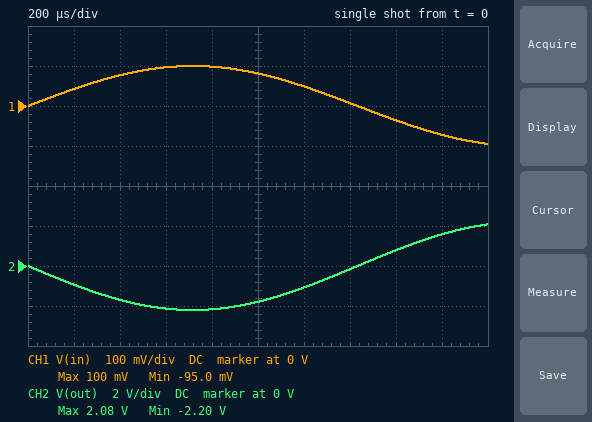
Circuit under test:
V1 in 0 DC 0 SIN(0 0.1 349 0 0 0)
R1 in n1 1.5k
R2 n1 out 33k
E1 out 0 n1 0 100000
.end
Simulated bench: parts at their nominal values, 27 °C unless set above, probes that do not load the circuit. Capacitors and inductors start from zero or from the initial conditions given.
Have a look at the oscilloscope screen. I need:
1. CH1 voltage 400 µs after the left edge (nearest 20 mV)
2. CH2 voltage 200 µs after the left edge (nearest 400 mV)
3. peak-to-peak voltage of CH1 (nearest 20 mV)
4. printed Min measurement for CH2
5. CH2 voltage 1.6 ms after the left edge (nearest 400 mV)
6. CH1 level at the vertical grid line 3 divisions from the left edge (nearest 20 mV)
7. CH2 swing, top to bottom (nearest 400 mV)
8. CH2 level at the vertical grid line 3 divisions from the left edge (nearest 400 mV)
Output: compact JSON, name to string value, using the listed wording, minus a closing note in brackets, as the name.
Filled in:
{"CH1 voltage 400 µs after the left edge": "80 mV", "CH2 voltage 200 µs after the left edge": "-800 mV", "peak-to-peak voltage of CH1": "200 mV", "printed Min measurement for CH2": "-2.20 V", "CH2 voltage 1.6 ms after the left edge": "800 mV", "CH1 level at the vertical grid line 3 divisions from the left edge": "100 mV", "CH2 swing, top to bottom": "4.4 V", "CH2 level at the vertical grid line 3 divisions from the left edge": "-2.0 V"}
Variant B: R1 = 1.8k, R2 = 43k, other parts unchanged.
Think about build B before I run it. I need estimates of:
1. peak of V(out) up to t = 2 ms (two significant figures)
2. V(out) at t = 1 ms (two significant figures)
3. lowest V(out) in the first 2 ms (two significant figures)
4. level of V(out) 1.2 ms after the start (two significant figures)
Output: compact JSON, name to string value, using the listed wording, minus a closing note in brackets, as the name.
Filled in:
{"peak of V(out) up to t = 2 ms": "2.3 V", "V(out) at t = 1 ms": "-1.9 V", "lowest V(out) in the first 2 ms": "-2.4 V", "level of V(out) 1.2 ms after the start": "-1.2 V"}
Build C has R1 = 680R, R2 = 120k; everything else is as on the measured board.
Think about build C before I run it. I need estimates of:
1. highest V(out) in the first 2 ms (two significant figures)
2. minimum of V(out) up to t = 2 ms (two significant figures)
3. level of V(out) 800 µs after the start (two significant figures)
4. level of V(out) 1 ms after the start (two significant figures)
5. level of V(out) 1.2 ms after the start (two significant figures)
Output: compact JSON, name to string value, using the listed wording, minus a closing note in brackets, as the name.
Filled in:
{"highest V(out) in the first 2 ms": "17 V", "minimum of V(out) up to t = 2 ms": "-18 V", "level of V(out) 800 µs after the start": "-17 V", "level of V(out) 1 ms after the start": "-14 V", "level of V(out) 1.2 ms after the start": "-8.6 V"}
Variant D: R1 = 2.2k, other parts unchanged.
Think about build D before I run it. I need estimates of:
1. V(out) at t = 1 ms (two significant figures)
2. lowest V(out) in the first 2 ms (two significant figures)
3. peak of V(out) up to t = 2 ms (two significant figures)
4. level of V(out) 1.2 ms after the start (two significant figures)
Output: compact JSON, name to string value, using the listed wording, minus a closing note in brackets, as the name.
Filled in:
{"V(out) at t = 1 ms": "-1.2 V", "lowest V(out) in the first 2 ms": "-1.5 V", "peak of V(out) up to t = 2 ms": "1.4 V", "level of V(out) 1.2 ms after the start": "-730 mV"}
